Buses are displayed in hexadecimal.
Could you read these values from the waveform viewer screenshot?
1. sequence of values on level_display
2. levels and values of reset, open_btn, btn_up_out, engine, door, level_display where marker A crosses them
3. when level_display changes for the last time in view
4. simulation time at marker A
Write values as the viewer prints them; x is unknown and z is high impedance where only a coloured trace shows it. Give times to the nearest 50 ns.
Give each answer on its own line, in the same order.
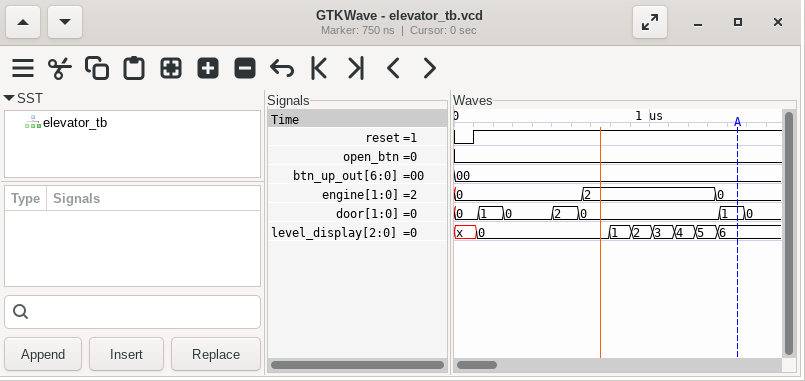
x, 0, 1, 2, 3, 4, 5, 6
reset=1, open_btn=0, btn_up_out=00, engine=0, door=1, level_display=6
1350 ns
1450 ns
